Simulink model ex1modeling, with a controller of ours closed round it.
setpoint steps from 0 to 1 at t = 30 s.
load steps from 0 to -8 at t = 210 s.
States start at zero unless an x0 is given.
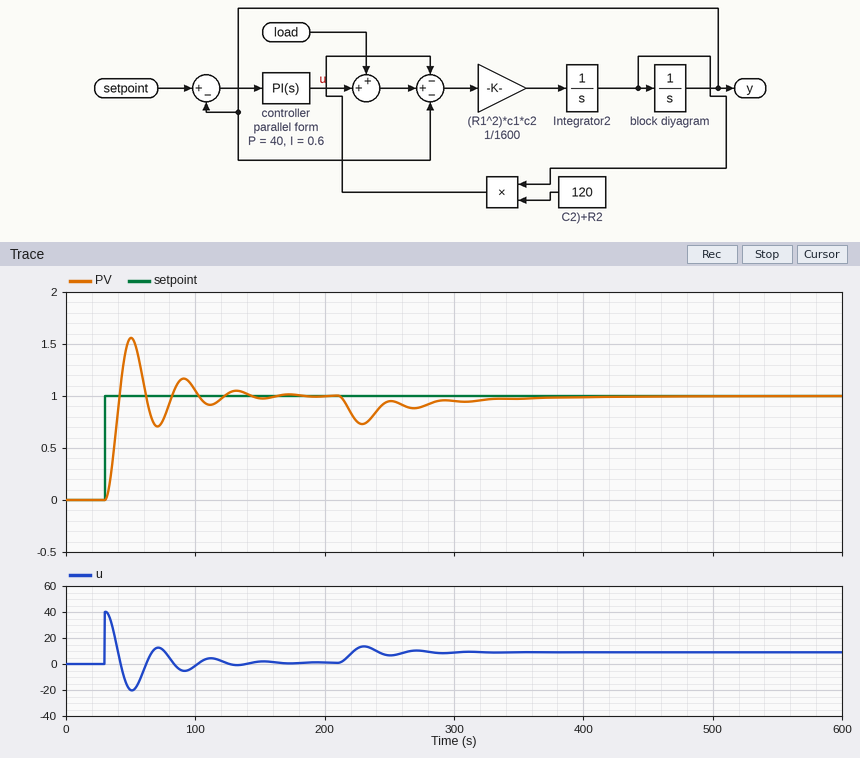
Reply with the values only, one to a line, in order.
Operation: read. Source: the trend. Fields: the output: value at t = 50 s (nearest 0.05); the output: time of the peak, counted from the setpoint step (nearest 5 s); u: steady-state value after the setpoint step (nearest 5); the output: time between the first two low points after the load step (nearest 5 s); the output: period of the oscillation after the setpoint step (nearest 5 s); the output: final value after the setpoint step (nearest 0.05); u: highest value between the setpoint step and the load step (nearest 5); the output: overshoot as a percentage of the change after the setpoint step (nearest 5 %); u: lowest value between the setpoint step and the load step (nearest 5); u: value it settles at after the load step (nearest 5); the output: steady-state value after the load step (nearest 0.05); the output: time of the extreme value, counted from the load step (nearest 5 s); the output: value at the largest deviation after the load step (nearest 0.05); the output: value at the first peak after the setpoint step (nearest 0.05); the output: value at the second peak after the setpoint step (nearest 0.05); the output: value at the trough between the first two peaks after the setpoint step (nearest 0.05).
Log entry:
1.55
20 s
0
40 s
40 s
1.00
40
55 %
-20
10
1.00
20 s
0.75
1.55
1.15
0.70
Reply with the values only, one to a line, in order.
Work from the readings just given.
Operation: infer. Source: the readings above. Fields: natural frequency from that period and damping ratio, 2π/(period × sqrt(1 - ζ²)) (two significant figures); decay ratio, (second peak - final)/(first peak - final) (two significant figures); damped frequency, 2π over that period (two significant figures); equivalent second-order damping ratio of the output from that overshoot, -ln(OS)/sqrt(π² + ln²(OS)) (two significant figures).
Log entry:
0.16 rad/s
0.27
0.16 rad/s
0.19
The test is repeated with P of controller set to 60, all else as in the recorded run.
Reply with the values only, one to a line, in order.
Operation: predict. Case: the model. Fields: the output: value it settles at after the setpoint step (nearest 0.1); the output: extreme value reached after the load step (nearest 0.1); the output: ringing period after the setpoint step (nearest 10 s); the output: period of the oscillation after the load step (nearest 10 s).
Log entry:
1.0
0.8
30 s
30 s
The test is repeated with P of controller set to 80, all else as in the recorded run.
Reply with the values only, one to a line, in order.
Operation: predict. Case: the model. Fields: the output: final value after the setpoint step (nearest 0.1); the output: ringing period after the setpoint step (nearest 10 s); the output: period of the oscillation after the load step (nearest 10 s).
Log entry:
1.0
30 s
30 s
